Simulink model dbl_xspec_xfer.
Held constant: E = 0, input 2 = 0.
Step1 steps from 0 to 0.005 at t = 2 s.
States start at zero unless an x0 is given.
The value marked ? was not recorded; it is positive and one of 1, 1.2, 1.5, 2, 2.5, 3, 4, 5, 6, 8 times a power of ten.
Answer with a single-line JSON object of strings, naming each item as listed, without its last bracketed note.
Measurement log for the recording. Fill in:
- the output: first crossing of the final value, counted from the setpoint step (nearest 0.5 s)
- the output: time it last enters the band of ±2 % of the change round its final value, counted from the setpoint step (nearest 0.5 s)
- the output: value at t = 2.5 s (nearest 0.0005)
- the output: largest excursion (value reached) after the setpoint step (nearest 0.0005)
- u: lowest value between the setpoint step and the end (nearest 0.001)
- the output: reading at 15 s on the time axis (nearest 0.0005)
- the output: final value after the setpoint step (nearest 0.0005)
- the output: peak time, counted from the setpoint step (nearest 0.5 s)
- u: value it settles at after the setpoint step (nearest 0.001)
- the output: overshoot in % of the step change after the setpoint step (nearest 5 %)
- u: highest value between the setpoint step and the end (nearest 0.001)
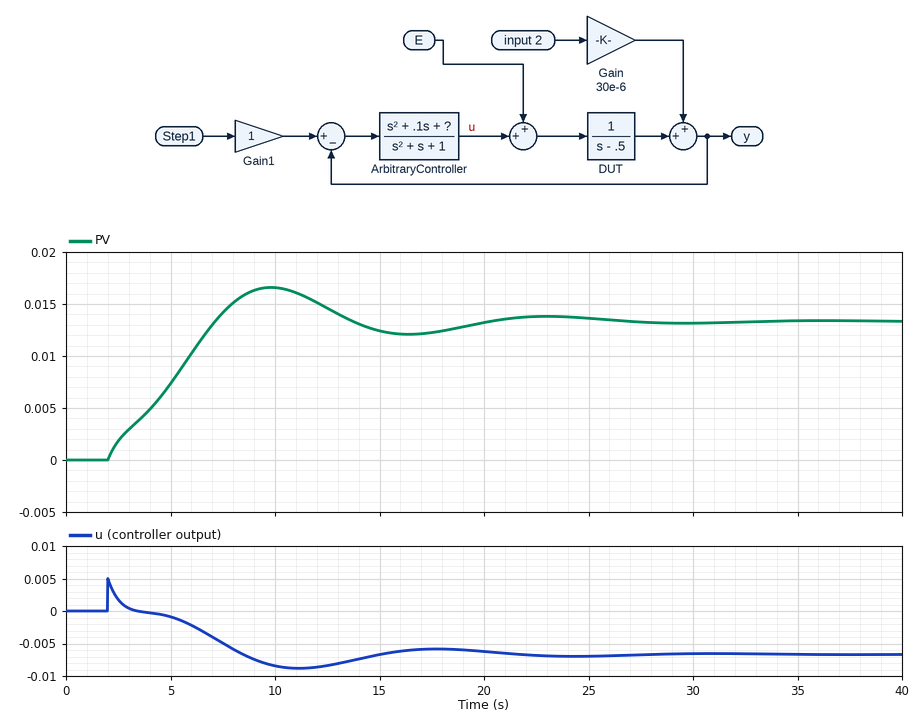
{"the output: first crossing of the final value, counted from the setpoint step": "5.0 s", "the output: time it last enters the band of ±2 % of the change round its final value, counted from the setpoint step": "23.0 s", "the output: value at t = 2.5 s": "0.0020", "the output: largest excursion (value reached) after the setpoint step": "0.0165", "u: lowest value between the setpoint step and the end": "-0.009", "the output: reading at 15 s on the time axis": "0.0125", "the output: final value after the setpoint step": "0.0135", "the output: peak time, counted from the setpoint step": "8.0 s", "u: value it settles at after the setpoint step": "-0.007", "the output: overshoot in % of the step change after the setpoint step": "25 %", "u: highest value between the setpoint step and the end": "0.005"}
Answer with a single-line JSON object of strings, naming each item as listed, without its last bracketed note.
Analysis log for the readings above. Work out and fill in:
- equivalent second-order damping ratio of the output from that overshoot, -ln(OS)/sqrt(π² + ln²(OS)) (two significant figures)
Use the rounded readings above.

{"equivalent second-order damping ratio of the output from that overshoot, -ln(OS)/sqrt(π² + ln²(OS))": "0.40"}
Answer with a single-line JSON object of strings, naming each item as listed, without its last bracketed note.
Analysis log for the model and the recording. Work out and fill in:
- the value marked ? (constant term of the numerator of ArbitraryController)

{"the value marked ?": "0.8"}
